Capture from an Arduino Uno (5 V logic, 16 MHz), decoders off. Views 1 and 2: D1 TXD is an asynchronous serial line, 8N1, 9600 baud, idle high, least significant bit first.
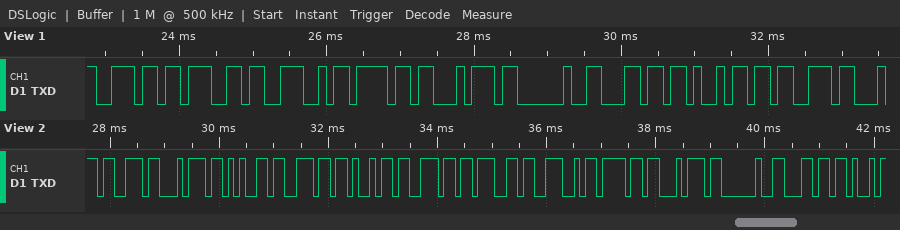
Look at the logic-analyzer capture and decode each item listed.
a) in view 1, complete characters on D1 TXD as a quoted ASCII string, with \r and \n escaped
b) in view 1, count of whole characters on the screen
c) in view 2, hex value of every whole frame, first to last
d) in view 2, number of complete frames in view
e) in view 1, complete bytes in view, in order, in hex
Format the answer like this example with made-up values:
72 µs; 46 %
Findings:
"ngNot lis"; 9; 0x73 0x74 0x65 0x6E 0x69 0x6E 0x67 0x4E 0x6F 0x74 0x20 0x6C; 12; 0x6E 0x67 0x4E 0x6F 0x74 0x20 0x6C 0x69 0x73
